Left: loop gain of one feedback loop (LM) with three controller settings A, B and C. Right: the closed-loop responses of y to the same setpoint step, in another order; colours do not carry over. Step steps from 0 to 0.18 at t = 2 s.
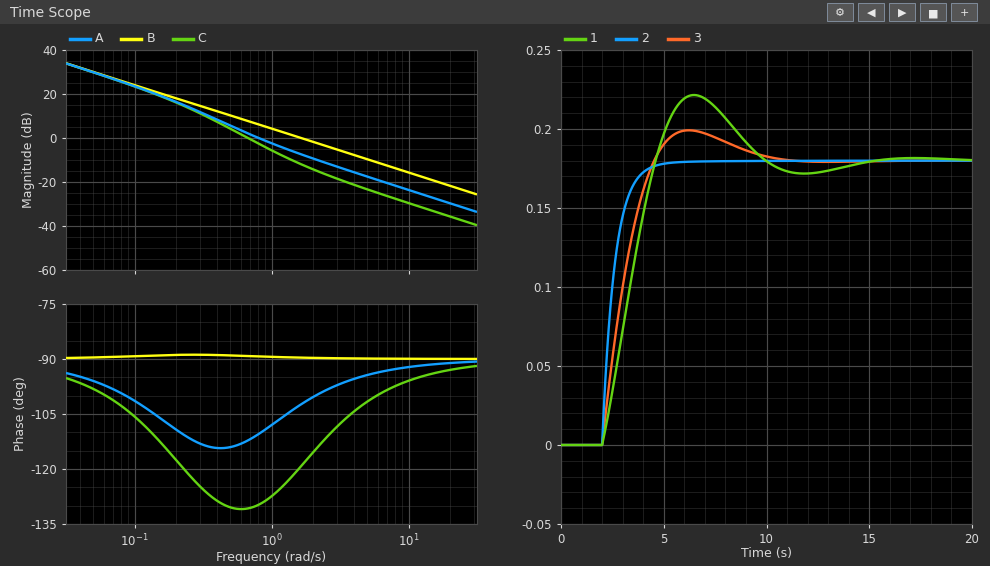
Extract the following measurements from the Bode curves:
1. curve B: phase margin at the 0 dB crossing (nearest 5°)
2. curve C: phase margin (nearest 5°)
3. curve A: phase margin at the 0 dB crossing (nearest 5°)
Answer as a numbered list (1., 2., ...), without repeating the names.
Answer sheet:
1. 90°
2. 50°
3. 70°
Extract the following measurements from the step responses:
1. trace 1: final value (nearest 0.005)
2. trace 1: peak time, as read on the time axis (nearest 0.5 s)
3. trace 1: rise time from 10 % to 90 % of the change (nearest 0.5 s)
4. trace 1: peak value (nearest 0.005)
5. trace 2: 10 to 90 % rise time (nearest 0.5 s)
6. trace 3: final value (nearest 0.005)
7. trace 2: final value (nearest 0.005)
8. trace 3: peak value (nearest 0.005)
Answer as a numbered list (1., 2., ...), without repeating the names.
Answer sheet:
1. 0.180
2. 6.5 s
3. 2.0 s
4. 0.220
5. 1.5 s
6. 0.180
7. 0.180
8. 0.200
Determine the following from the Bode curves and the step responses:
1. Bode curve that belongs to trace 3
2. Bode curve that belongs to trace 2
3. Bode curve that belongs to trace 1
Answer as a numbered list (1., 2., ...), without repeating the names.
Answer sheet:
1. A
2. B
3. C
